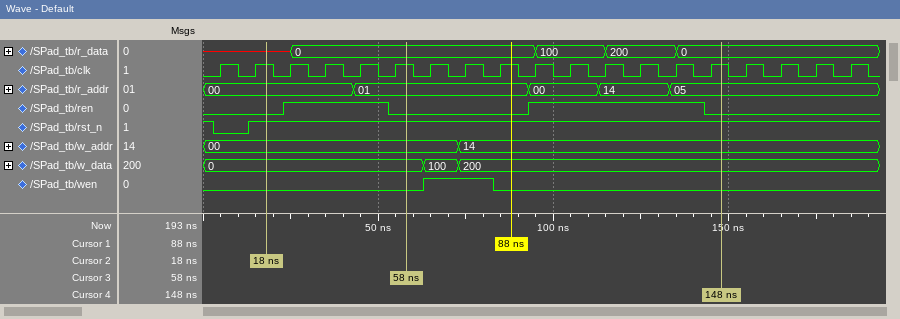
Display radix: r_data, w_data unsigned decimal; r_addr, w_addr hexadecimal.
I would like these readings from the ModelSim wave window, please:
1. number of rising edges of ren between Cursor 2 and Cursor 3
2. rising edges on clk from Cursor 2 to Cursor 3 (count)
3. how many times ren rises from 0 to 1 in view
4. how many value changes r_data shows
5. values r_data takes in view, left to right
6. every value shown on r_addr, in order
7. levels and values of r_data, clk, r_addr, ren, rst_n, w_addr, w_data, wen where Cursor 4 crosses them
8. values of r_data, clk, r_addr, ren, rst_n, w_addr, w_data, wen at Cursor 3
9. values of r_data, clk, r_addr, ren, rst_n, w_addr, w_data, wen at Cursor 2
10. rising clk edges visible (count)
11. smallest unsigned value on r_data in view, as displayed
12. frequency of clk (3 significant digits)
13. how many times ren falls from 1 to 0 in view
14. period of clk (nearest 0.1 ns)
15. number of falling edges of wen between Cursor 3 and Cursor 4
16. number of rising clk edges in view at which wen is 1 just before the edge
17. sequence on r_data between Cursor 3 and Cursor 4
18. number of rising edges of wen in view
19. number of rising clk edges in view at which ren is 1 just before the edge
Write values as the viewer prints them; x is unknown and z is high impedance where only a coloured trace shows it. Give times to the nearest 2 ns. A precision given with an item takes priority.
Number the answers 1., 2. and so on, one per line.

1. 1
2. 4
3. 2
4. 4
5. x, 0, 100, 200, 0
6. 00, 01, 00, 14, 05
7. r_data=0, clk=1, r_addr=05, ren=0, rst_n=1, w_addr=14, w_data=200, wen=0
8. r_data=0, clk=1, r_addr=01, ren=0, rst_n=1, w_addr=00, w_data=0, wen=0
9. r_data=x, clk=1, r_addr=00, ren=0, rst_n=1, w_addr=00, w_data=0, wen=0
10. 19
11. 0
12. 100 MHz
13. 2
14. 10 ns
15. 1
16. 2
17. 0, 100, 200, 0
18. 1
19. 8
